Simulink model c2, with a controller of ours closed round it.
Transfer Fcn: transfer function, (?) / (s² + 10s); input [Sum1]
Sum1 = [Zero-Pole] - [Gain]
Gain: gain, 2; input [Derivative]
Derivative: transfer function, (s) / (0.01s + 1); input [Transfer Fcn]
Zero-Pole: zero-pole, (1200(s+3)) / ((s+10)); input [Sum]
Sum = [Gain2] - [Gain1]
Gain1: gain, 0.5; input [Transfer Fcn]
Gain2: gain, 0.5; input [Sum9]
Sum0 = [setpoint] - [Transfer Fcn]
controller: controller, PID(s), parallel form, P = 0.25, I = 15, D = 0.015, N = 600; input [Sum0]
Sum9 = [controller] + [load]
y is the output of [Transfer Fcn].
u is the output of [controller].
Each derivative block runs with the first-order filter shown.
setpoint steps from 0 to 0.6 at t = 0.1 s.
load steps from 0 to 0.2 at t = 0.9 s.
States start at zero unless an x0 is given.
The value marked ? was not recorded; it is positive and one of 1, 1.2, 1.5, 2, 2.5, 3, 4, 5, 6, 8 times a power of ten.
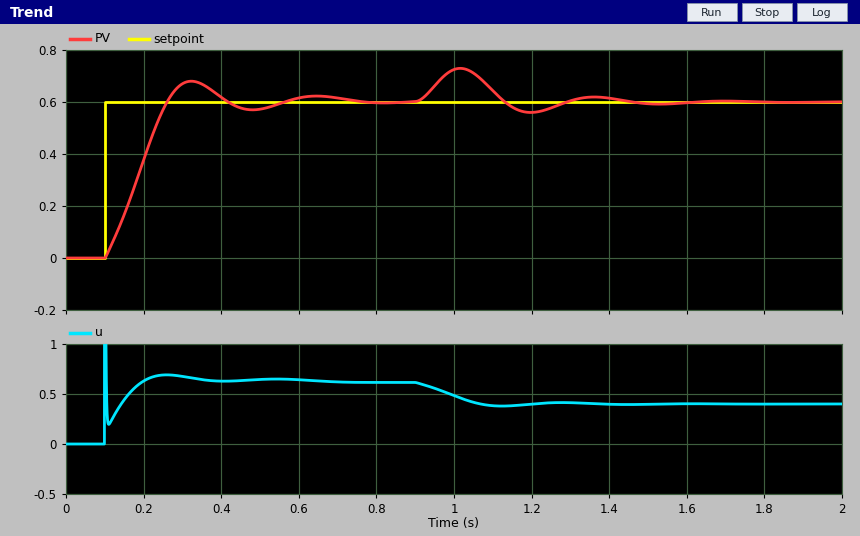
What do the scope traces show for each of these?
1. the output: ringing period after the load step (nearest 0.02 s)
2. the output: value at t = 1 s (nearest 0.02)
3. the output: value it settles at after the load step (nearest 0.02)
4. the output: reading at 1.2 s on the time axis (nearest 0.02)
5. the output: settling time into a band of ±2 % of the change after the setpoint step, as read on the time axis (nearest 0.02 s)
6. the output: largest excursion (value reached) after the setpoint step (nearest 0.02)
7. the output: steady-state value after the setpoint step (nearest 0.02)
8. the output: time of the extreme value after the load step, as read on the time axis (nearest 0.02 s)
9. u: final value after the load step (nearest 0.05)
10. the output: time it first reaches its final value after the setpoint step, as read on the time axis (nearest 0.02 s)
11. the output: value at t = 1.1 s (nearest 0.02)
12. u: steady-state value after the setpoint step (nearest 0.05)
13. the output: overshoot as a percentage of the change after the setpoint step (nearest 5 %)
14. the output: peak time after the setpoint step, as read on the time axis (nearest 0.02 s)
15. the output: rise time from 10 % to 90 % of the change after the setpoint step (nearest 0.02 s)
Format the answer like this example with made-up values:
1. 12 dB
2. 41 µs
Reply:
1. 0.34 s
2. 0.72
3. 0.60
4. 0.56
5. 0.72 s
6. 0.68
7. 0.60
8. 1.02 s
9. 0.40
10. 0.26 s
11. 0.64
12. 0.60
13. 15 %
14. 0.32 s
15. 0.12 s
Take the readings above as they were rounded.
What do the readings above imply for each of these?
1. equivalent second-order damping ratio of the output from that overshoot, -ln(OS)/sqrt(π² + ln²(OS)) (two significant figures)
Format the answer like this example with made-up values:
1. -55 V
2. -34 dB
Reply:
1. 0.52
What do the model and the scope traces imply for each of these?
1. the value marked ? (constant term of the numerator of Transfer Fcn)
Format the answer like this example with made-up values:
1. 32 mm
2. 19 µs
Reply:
1. 0.6
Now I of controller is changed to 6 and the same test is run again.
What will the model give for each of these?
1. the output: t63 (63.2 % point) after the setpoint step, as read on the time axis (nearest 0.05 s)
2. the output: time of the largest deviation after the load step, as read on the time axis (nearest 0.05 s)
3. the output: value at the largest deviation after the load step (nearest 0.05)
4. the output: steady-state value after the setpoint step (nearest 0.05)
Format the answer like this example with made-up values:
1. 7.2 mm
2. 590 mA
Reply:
1. 0.30 s
2. 1.05 s
3. 0.75
4. 0.60
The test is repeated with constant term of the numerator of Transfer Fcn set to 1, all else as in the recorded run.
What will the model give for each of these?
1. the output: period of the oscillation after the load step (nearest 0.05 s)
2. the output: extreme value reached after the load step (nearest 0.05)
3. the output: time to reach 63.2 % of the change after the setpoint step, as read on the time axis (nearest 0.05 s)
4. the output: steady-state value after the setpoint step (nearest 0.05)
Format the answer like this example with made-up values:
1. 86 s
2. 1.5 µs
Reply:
1. 0.25 s
2. 0.75
3. 0.20 s
4. 0.60
